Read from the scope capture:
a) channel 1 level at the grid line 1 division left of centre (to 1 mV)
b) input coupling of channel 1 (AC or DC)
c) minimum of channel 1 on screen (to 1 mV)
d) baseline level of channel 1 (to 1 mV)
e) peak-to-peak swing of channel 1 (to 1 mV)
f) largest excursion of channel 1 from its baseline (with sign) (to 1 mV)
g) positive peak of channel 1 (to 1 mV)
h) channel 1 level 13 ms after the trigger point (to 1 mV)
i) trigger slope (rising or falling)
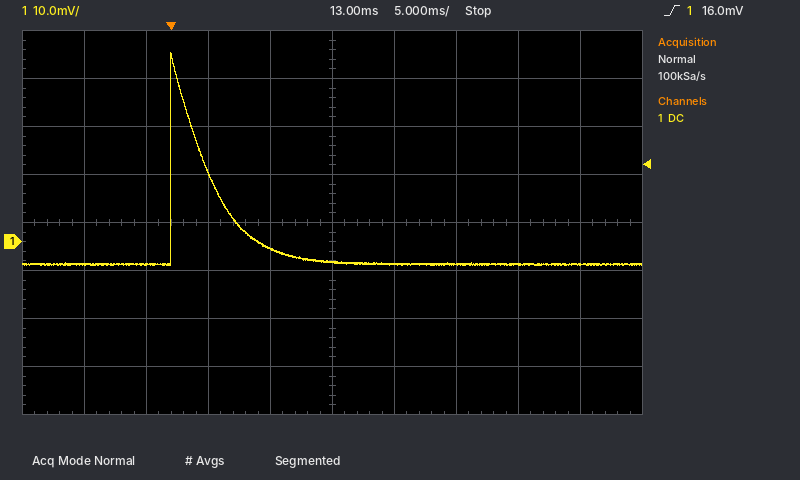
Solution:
-1 mV
DC
-5 mV
-5 mV
44 mV
+44 mV
39 mV
-4 mV
rising
